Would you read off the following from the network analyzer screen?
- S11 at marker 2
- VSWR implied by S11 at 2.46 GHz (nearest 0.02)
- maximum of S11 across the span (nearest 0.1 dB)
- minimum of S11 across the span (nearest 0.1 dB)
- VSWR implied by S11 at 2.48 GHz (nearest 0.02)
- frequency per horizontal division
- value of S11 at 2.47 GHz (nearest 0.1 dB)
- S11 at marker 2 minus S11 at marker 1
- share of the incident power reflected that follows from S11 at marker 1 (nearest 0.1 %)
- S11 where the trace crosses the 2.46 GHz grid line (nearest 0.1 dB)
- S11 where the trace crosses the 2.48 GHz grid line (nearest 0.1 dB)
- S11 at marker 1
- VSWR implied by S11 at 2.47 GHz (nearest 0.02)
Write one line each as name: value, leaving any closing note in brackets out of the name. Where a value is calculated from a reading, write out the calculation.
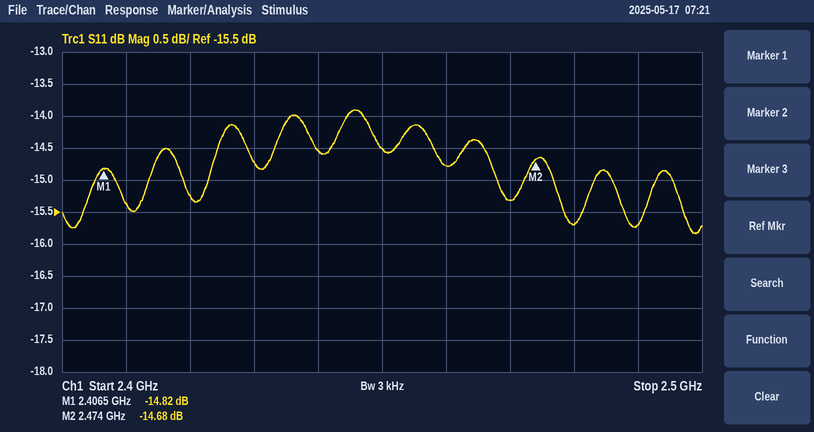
S11 at marker 2: -14.68 dB
VSWR implied by S11 at 2.46 GHz: |Γ| = 10^(-14.8/20) = 0.1820; VSWR = (1 + 0.1820)/(1 − 0.1820) ≈ 1.44
maximum of S11 across the span: -13.9 dB
minimum of S11 across the span: -15.8 dB
VSWR implied by S11 at 2.48 GHz: |Γ| = 10^(-15.7/20) = 0.1641; VSWR = (1 + 0.1641)/(1 − 0.1641) ≈ 1.39, so 1.40 to the nearest 0.02
frequency per horizontal division: 10 MHz
value of S11 at 2.47 GHz: -15.3 dB
S11 at marker 2 minus S11 at marker 1: -14.68 − (-14.82) = 0.14 dB
share of the incident power reflected that follows from S11 at marker 1: 10^(-14.82/10) ≈ 3.3 %
S11 where the trace crosses the 2.46 GHz grid line: -14.8 dB
S11 where the trace crosses the 2.48 GHz grid line: -15.7 dB
S11 at marker 1: -14.82 dB
VSWR implied by S11 at 2.47 GHz: |Γ| = 10^(-15.3/20) = 0.1718; VSWR = (1 + 0.1718)/(1 − 0.1718) ≈ 1.41, so 1.42 to the nearest 0.02
